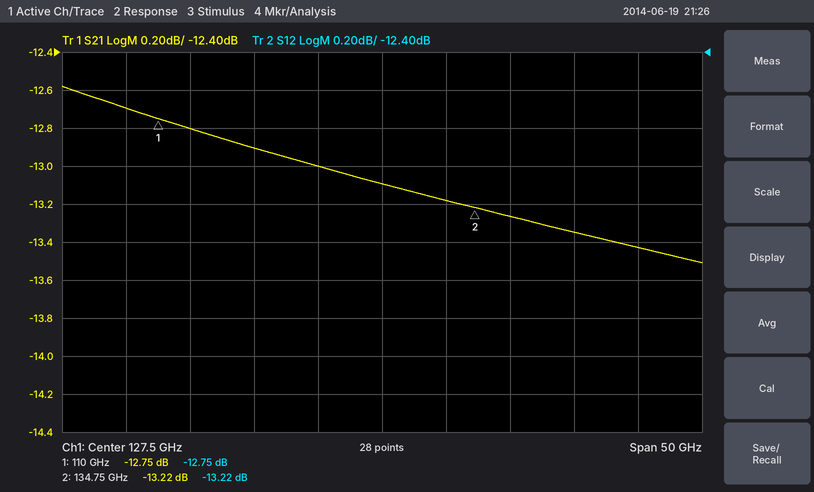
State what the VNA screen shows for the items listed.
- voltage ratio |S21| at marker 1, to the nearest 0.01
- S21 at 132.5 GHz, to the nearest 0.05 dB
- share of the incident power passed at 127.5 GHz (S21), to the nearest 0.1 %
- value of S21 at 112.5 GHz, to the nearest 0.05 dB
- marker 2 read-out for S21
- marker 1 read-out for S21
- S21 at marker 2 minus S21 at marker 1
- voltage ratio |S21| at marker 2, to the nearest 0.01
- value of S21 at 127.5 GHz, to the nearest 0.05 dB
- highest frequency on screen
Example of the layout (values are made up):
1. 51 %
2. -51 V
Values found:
1. 0.23
2. -13.20 dB
3. 4.9 %
4. -12.80 dB
5. -13.22 dB
6. -12.75 dB
7. -0.47 dB
8. 0.22
9. -13.10 dB
10. 152.5 GHz
